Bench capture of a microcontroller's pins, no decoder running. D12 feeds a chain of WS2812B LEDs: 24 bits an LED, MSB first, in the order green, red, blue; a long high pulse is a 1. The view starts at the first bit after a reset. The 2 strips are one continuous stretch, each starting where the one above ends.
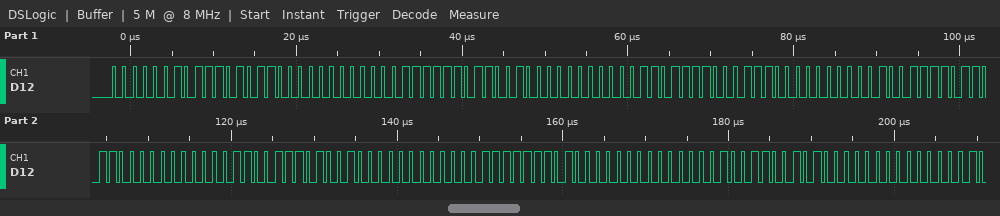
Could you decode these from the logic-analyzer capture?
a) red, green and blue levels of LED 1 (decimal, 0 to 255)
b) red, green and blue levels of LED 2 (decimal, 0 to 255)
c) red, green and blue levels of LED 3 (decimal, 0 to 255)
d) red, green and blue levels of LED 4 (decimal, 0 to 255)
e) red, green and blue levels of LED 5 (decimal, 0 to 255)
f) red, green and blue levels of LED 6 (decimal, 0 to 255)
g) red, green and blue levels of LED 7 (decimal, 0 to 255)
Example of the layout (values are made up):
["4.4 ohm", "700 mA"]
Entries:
["235, 2, 0", "217, 15, 0", "199, 27, 0", "182, 39, 0", "164, 51, 0", "160, 63, 0", "160, 76, 0"]
